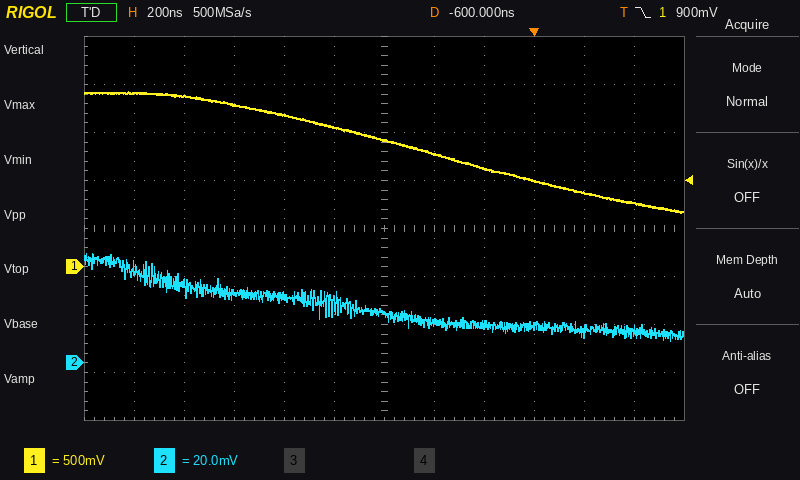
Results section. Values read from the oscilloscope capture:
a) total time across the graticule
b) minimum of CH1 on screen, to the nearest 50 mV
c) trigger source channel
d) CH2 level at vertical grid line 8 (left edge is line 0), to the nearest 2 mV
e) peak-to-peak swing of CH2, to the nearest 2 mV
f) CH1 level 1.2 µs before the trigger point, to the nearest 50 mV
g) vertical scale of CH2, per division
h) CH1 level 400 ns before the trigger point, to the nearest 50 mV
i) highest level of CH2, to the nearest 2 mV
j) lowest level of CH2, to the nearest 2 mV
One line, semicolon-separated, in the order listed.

2.4 µs; 550 mV; CH1; 16 mV; 36 mV; 1.70 V; 20 mV; 1.20 V; 46 mV; 10 mV
